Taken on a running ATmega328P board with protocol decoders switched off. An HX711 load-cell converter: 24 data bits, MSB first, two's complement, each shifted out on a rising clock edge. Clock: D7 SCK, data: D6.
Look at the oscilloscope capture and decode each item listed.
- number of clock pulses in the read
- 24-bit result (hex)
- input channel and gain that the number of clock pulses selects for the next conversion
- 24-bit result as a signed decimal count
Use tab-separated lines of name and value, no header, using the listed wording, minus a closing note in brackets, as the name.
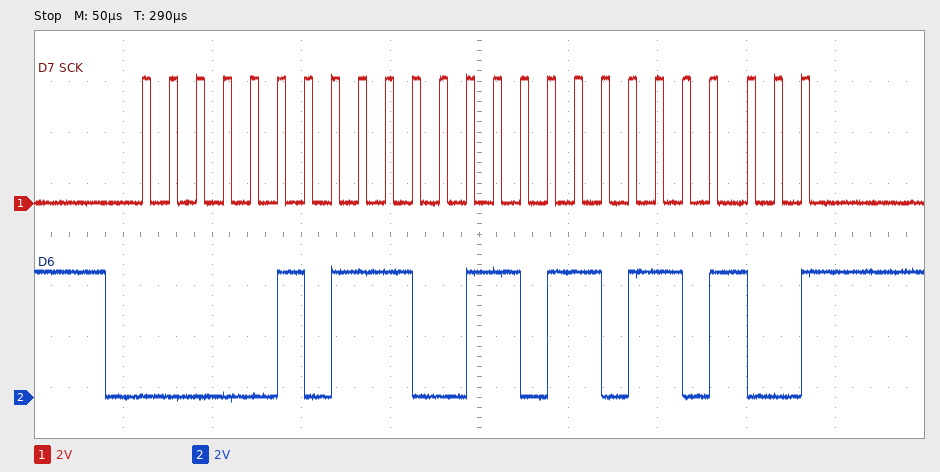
number of clock pulses in the read	25
24-bit result	0x05CDB4
input channel and gain that the number of clock pulses selects for the next conversion	channel A, gain 128
24-bit result as a signed decimal count	380340
